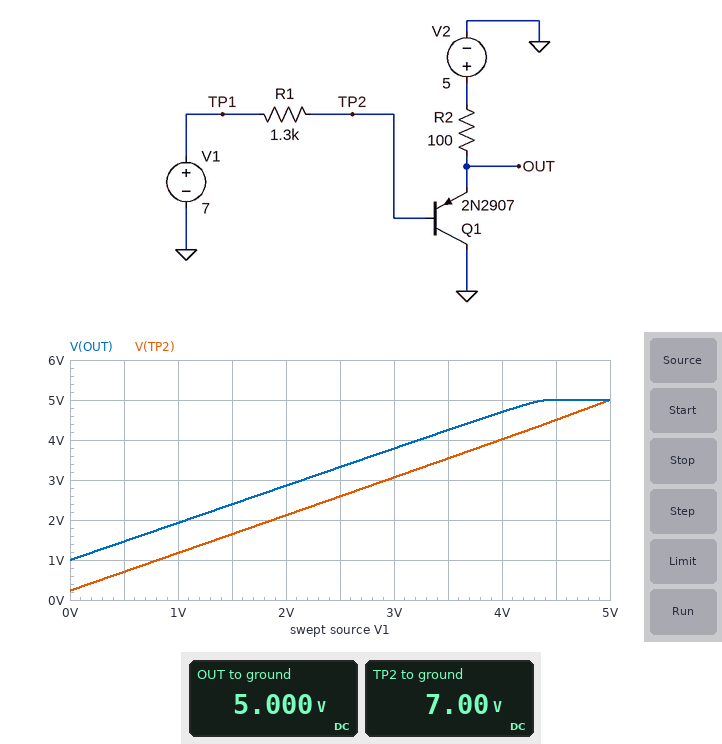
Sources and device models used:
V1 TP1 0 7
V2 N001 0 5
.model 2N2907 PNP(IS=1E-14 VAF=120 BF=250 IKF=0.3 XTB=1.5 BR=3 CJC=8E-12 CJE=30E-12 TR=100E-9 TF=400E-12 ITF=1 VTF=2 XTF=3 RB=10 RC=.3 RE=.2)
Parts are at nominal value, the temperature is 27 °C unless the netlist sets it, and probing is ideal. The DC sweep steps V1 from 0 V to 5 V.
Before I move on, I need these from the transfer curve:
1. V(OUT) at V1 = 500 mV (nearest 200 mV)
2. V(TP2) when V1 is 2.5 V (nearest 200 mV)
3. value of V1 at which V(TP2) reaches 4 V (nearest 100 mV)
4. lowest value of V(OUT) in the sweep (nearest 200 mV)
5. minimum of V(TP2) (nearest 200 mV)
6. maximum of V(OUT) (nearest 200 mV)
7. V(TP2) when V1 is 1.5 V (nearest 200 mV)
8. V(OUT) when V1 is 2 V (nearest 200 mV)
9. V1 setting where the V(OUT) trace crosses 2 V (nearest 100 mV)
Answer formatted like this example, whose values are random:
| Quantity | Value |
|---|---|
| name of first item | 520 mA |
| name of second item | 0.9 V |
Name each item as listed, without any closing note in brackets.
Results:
| Quantity | Value |
|---|---|
| V(OUT) at V1 = 500 mV | 1.4 V |
| V(TP2) when V1 is 2.5 V | 2.6 V |
| value of V1 at which V(TP2) reaches 4 V | 4.0 V |
| lowest value of V(OUT) in the sweep | 1.0 V |
| minimum of V(TP2) | 200 mV |
| maximum of V(OUT) | 5.0 V |
| V(TP2) when V1 is 1.5 V | 1.6 V |
| V(OUT) when V1 is 2 V | 2.8 V |
| V1 setting where the V(OUT) trace crosses 2 V | 1.1 V |
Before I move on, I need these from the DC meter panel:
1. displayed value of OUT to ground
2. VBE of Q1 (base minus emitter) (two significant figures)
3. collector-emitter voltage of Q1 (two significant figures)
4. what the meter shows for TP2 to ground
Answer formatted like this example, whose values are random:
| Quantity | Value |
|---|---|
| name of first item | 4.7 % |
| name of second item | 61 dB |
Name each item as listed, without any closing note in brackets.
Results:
| Quantity | Value |
|---|---|
| displayed value of OUT to ground | 5.000 V |
| VBE of Q1 (base minus emitter) | 2.0 V |
| collector-emitter voltage of Q1 | -5.0 V |
| what the meter shows for TP2 to ground | 7.00 V |
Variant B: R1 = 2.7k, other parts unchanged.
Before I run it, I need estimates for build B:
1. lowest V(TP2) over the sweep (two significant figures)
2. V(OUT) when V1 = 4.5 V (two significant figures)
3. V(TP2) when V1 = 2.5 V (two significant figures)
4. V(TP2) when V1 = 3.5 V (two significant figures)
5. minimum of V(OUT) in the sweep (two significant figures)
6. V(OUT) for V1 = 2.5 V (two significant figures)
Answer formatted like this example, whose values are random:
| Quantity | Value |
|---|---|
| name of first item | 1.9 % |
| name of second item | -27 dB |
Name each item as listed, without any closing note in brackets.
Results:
| Quantity | Value |
|---|---|
| lowest V(TP2) over the sweep | 460 mV |
| V(OUT) when V1 = 4.5 V | 5.0 V |
| V(TP2) when V1 = 2.5 V | 2.7 V |
| V(TP2) when V1 = 3.5 V | 3.6 V |
| minimum of V(OUT) in the sweep | 1.2 V |
| V(OUT) for V1 = 2.5 V | 3.4 V |
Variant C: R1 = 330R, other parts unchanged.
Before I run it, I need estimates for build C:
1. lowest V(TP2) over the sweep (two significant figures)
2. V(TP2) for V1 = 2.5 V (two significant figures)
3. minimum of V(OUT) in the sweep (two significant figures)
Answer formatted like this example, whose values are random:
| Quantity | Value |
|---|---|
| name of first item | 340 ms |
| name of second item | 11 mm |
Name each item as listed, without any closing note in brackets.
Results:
| Quantity | Value |
|---|---|
| lowest V(TP2) over the sweep | 62 mV |
| V(TP2) for V1 = 2.5 V | 2.5 V |
| minimum of V(OUT) in the sweep | 830 mV |
